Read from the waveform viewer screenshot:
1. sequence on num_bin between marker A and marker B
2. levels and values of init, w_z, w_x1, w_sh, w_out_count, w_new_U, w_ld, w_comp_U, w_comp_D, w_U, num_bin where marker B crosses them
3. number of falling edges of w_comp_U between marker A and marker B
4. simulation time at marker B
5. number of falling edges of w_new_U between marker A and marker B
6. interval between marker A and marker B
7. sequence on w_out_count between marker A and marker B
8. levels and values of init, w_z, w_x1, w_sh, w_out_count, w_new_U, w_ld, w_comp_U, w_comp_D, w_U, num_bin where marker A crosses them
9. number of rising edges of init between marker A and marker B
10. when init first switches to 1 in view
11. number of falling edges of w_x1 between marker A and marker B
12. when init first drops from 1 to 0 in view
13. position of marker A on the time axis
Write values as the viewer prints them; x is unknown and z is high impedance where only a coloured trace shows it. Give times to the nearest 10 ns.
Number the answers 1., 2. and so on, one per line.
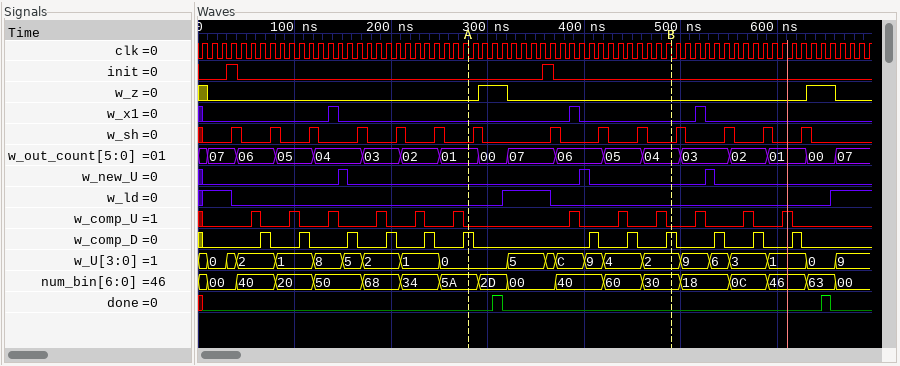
1. 5A, 2D, 00, 40, 60, 30
2. init=0, w_z=0, w_x1=0, w_sh=0, w_out_count=04, w_new_U=0, w_ld=0, w_comp_U=0, w_comp_D=1, w_U=2, num_bin=30
3. 3
4. 490 ns
5. 1
6. 210 ns
7. 01, 00, 07, 06, 05, 04
8. init=0, w_z=0, w_x1=0, w_sh=0, w_out_count=01, w_new_U=0, w_ld=0, w_comp_U=0, w_comp_D=1, w_U=0, num_bin=5A
9. 1
10. 30 ns
11. 1
12. 40 ns
13. 280 ns
